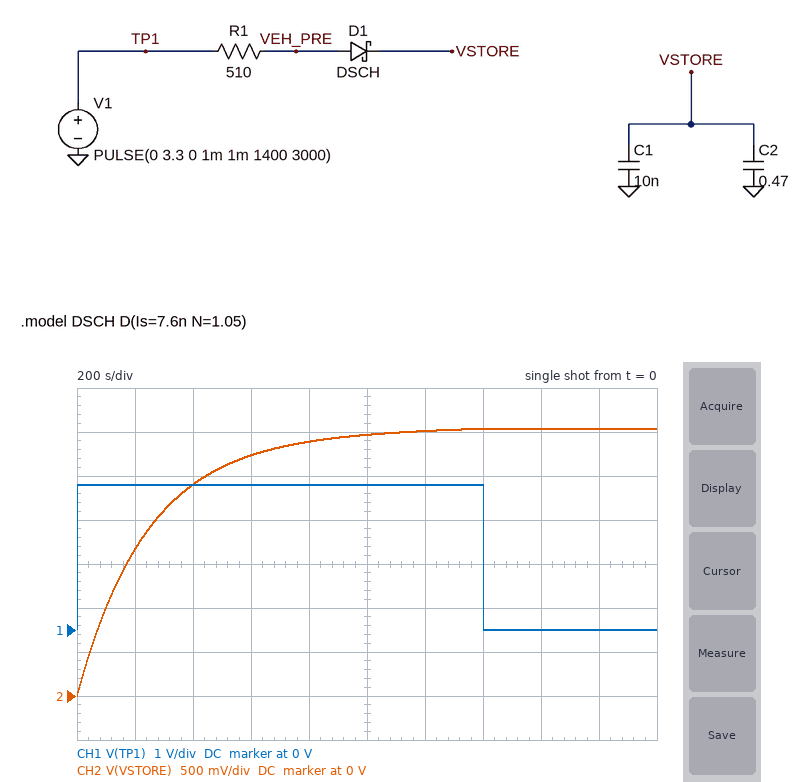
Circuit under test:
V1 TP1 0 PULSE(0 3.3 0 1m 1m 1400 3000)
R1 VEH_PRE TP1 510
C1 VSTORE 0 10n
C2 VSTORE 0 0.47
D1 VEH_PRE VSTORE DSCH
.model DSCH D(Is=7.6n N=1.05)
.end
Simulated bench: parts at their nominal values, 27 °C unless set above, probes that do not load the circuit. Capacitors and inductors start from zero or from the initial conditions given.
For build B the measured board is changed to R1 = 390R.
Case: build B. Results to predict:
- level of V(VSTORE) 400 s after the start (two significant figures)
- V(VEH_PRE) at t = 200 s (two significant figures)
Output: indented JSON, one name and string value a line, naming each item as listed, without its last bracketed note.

{
  "level of V(VSTORE) 400 s after the start": "2.6 V",
  "V(VEH_PRE) at t = 200 s": "2.3 V"
}
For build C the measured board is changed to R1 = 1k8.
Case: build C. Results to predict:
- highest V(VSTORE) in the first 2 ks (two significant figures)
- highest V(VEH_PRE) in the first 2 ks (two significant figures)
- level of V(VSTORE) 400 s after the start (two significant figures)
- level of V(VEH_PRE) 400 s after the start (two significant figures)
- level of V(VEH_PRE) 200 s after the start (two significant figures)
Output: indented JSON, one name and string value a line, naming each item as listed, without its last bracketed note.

{
  "highest V(VSTORE) in the first 2 ks": "2.4 V",
  "highest V(VEH_PRE) in the first 2 ks": "2.7 V",
  "level of V(VSTORE) 400 s after the start": "1.1 V",
  "level of V(VEH_PRE) 400 s after the start": "1.4 V",
  "level of V(VEH_PRE) 200 s after the start": "950 mV"
}
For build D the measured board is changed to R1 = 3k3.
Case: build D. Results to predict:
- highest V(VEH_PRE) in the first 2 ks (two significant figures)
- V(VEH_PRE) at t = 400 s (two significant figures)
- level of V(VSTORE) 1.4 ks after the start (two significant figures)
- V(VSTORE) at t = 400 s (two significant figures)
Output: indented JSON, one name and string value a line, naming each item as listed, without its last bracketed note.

{
  "highest V(VEH_PRE) in the first 2 ks": "2.1 V",
  "V(VEH_PRE) at t = 400 s": "990 mV",
  "level of V(VSTORE) 1.4 ks after the start": "1.8 V",
  "V(VSTORE) at t = 400 s": "680 mV"
}
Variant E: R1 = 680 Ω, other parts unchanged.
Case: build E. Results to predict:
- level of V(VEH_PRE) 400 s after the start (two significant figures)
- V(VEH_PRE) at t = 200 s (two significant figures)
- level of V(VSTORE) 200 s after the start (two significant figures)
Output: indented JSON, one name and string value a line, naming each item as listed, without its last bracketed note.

{
  "level of V(VEH_PRE) 400 s after the start": "2.4 V",
  "V(VEH_PRE) at t = 200 s": "1.7 V",
  "level of V(VSTORE) 200 s after the start": "1.4 V"
}
